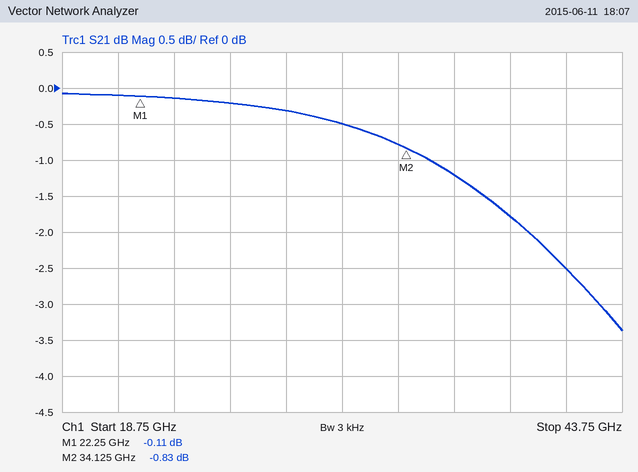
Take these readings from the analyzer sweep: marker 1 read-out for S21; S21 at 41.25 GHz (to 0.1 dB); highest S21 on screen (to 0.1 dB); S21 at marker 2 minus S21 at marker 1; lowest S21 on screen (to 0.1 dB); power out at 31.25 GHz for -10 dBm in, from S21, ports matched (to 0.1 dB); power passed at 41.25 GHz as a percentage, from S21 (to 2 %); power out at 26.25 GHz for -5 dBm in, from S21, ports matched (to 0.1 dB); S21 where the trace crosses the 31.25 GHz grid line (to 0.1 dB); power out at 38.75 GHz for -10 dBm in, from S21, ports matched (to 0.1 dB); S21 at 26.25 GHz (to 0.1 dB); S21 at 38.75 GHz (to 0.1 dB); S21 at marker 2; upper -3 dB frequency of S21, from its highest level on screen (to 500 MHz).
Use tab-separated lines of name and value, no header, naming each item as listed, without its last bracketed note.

marker 1 read-out for S21	-0.11 dB
S21 at 41.25 GHz	-2.5 dB
highest S21 on screen	-0.1 dB
S21 at marker 2 minus S21 at marker 1	-0.72 dB
lowest S21 on screen	-3.4 dB
power out at 31.25 GHz for -10 dBm in, from S21, ports matched	-10.5 dBm
power passed at 41.25 GHz as a percentage, from S21	56 %
power out at 26.25 GHz for -5 dBm in, from S21, ports matched	-5.2 dBm
S21 where the trace crosses the 31.25 GHz grid line	-0.5 dB
power out at 38.75 GHz for -10 dBm in, from S21, ports matched	-11.8 dBm
S21 at 26.25 GHz	-0.2 dB
S21 at 38.75 GHz	-1.8 dB
S21 at marker 2	-0.83 dB
upper -3 dB frequency of S21, from its highest level on screen	43.0 GHz
